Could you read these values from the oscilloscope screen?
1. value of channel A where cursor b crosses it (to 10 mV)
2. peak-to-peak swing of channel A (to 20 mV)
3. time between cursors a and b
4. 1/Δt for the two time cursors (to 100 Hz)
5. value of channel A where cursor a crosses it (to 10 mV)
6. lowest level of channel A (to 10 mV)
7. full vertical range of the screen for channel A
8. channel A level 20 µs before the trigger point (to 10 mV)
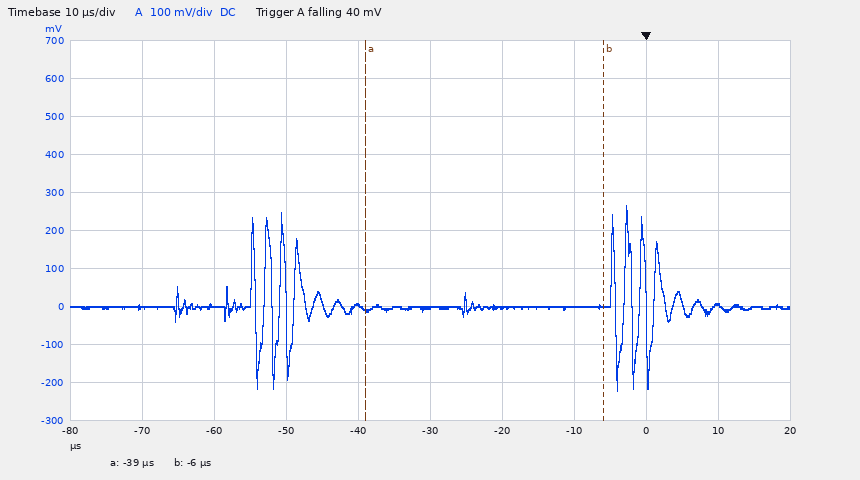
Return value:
0 mV
480 mV
33 µs
30.3 kHz
-10 mV
-220 mV
1 V
0 mV
